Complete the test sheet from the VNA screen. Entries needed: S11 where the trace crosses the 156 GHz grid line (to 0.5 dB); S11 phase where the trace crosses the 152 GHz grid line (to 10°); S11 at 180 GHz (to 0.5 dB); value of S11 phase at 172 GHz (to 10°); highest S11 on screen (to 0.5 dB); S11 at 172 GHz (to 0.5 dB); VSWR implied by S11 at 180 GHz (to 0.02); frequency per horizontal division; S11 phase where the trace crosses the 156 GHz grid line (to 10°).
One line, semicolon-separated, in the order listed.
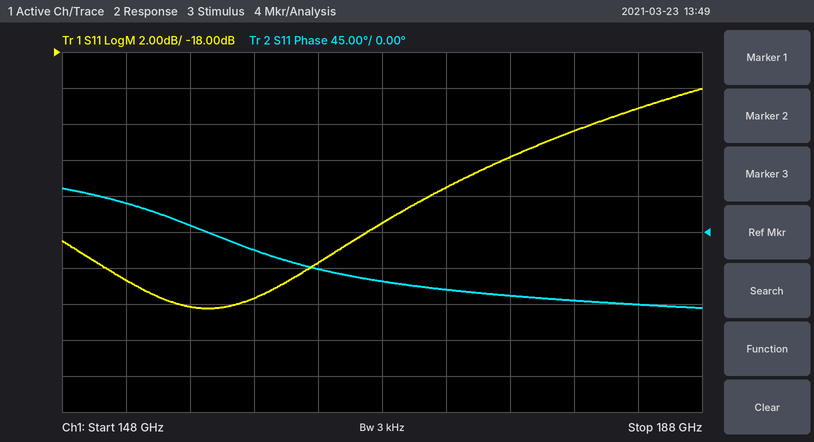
-32.0 dB; 40°; -22.5 dB; -70°; -20.0 dB; -25.5 dB; 1.16; 4 GHz; 10°
